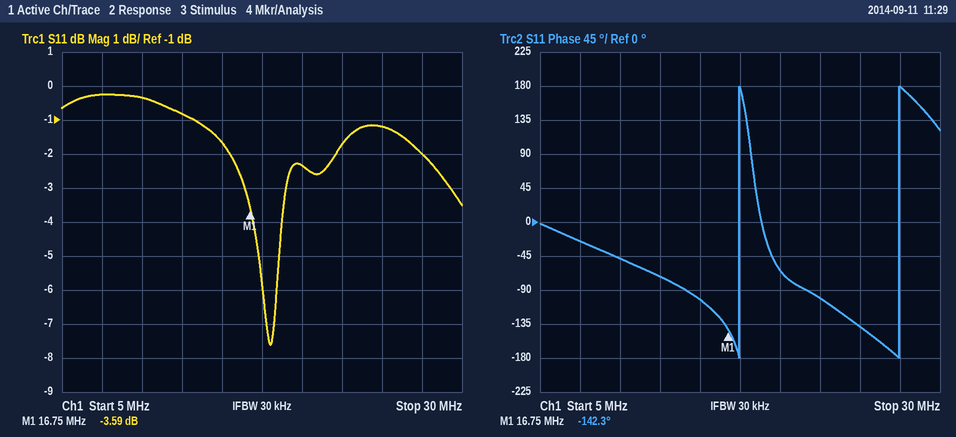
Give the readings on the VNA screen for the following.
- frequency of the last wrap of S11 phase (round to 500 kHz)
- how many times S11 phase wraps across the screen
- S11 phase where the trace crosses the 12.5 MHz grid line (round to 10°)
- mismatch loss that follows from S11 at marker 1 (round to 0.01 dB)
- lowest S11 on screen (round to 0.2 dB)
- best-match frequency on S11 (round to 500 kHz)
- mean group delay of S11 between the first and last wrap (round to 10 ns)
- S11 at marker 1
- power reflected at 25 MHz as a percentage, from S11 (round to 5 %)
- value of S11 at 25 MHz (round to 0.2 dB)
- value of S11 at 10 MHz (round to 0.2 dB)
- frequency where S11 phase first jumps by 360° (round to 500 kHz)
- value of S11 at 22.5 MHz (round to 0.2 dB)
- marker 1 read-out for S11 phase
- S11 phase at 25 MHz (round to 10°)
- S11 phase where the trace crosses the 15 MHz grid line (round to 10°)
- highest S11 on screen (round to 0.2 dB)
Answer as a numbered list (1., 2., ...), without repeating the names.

1. 27.5 MHz
2. 2
3. -70°
4. 2.50 dB
5. -7.6 dB
6. 18.0 MHz
7. 100 ns
8. -3.59 dB
9. 75 %
10. -1.2 dB
11. -0.4 dB
12. 17.5 MHz
13. -1.8 dB
14. -142.3°
15. -140°
16. -100°
17. -0.2 dB
